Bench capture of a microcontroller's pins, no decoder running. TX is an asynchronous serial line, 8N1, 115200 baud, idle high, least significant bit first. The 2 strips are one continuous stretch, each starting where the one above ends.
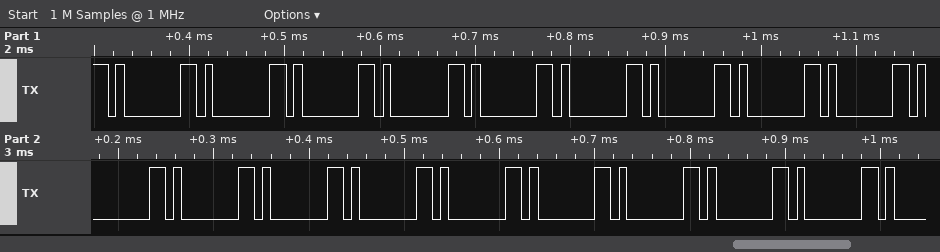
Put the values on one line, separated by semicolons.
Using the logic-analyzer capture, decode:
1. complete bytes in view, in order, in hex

0x01 0x01 0x01 0x01 0x01 0x01 0x01 0x01 0x01 0x01 0x01 0x01 0x01 0x01 0x01 0x01 0x01 0x01
